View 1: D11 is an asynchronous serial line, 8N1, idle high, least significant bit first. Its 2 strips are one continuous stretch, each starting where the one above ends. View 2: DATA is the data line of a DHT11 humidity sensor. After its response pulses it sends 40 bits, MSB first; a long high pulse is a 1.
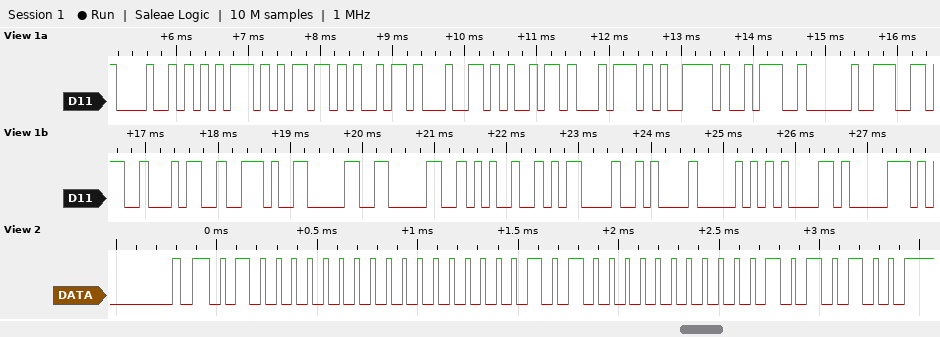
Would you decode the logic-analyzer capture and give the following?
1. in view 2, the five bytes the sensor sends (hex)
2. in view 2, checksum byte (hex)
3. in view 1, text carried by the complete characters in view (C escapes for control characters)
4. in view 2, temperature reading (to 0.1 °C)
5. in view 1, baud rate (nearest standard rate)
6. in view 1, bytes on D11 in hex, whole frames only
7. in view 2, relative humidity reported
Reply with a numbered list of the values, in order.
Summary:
1. 40 00 14 00 54
2. 0x54
3. "Humidity: 64.00%\r\nPap"
4. 20.0 °C
5. 9600 baud
6. 48 75 6D 69 64 69 74 79 3A 20 36 34 2E 30 30 25 0D 0A 50 61 70
7. 64 %
